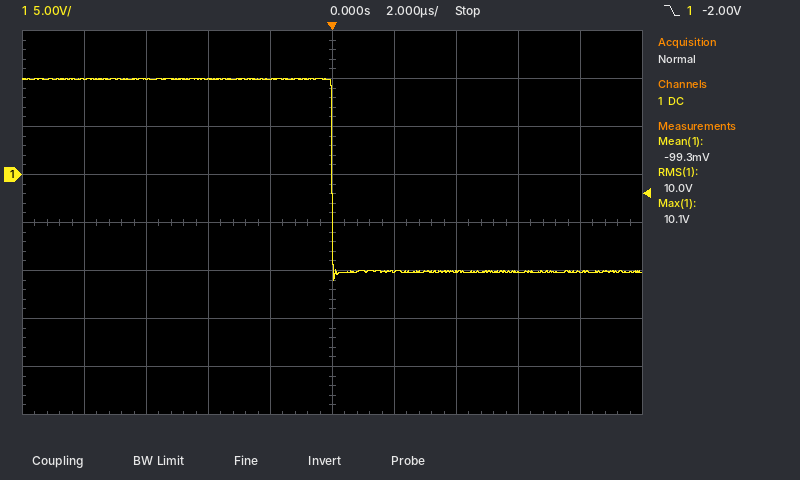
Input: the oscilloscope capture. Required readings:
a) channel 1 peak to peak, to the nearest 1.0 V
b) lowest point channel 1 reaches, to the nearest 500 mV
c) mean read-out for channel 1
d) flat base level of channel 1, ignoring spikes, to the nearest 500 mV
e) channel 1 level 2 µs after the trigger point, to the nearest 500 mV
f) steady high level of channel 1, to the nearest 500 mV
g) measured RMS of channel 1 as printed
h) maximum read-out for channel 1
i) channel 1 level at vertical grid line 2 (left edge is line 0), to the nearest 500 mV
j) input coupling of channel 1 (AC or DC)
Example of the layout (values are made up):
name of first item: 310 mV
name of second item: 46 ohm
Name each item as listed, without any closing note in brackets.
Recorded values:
channel 1 peak to peak, to the nearest 1.0 V: 21.0 V
lowest point channel 1 reaches, to the nearest 500 mV: -11.0 V
mean read-out for channel 1: -99.3 mV
flat base level of channel 1, ignoring spikes, to the nearest 500 mV: -10.0 V
channel 1 level 2 µs after the trigger point, to the nearest 500 mV: -10.0 V
steady high level of channel 1, to the nearest 500 mV: 10.0 V
measured RMS of channel 1 as printed: 10.0 V
maximum read-out for channel 1: 10.1 V
channel 1 level at vertical grid line 2 (left edge is line 0), to the nearest 500 mV: 10.0 V
input coupling of channel 1: DC
